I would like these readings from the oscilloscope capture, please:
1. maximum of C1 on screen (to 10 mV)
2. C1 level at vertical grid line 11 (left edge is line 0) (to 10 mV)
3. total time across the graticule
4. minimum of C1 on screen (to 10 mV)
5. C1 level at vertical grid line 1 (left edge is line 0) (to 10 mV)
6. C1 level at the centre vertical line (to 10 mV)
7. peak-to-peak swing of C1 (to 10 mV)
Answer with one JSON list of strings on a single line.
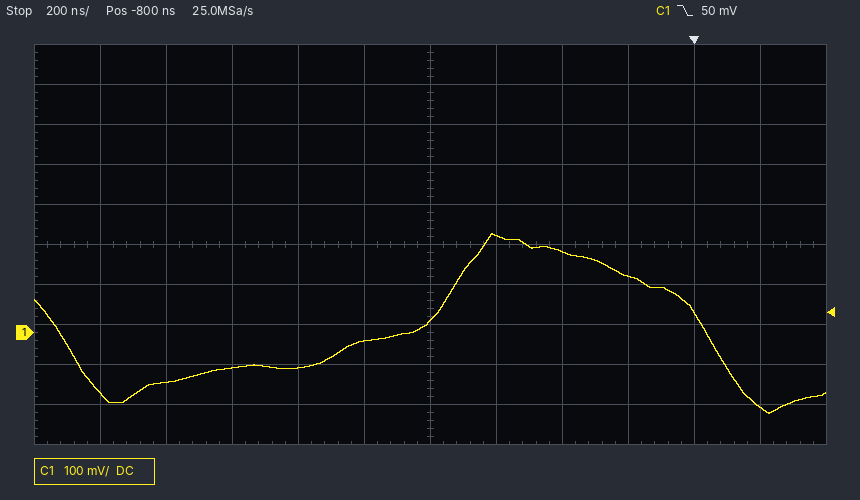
["250 mV", "-190 mV", "2.4 µs", "-200 mV", "-150 mV", "30 mV", "450 mV"]
